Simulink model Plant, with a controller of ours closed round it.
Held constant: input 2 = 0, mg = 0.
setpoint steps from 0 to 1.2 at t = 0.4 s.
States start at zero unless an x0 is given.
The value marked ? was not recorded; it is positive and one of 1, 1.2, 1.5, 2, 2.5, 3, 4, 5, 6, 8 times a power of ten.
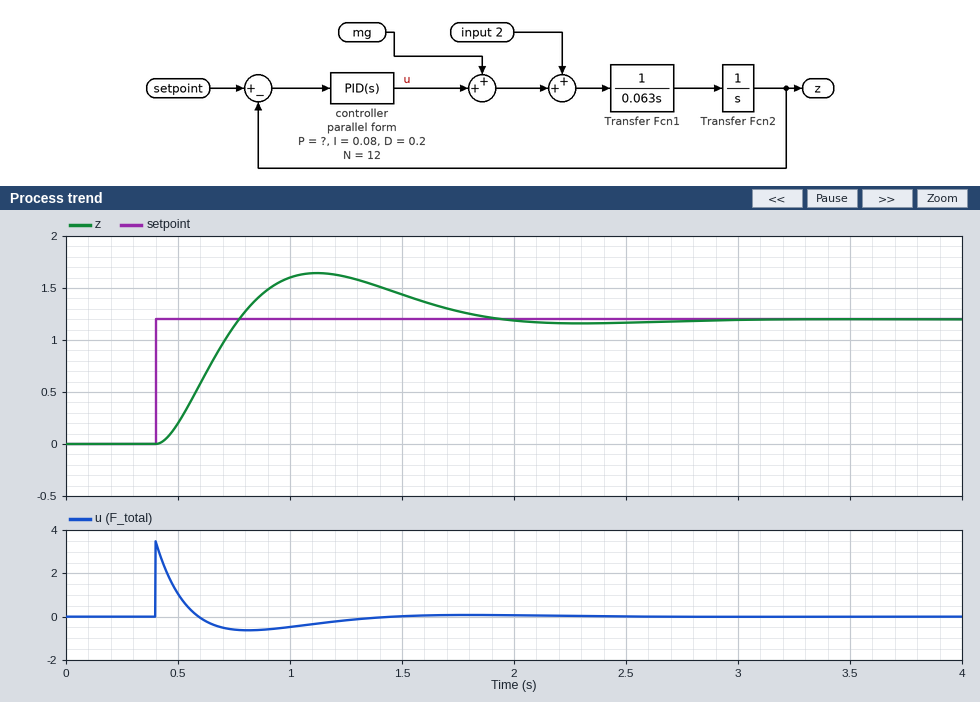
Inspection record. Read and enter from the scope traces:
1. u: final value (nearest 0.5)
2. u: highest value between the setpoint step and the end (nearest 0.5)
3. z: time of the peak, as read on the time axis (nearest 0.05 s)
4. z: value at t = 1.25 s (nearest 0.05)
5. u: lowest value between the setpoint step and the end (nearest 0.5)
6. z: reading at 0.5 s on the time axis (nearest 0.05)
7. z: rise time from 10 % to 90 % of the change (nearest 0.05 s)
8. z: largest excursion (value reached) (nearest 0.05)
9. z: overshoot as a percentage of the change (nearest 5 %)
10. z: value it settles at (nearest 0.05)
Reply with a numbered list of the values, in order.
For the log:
1. 0.0
2. 3.5
3. 1.10 s
4. 1.60
5. -0.5
6. 0.20
7. 0.25 s
8. 1.65
9. 35 %
10. 1.20
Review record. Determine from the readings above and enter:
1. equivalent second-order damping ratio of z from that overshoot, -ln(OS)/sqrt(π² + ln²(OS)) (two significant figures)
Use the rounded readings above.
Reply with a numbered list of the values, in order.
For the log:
1. 0.32
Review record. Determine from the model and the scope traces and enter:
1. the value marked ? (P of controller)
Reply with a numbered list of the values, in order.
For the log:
1. 0.5
